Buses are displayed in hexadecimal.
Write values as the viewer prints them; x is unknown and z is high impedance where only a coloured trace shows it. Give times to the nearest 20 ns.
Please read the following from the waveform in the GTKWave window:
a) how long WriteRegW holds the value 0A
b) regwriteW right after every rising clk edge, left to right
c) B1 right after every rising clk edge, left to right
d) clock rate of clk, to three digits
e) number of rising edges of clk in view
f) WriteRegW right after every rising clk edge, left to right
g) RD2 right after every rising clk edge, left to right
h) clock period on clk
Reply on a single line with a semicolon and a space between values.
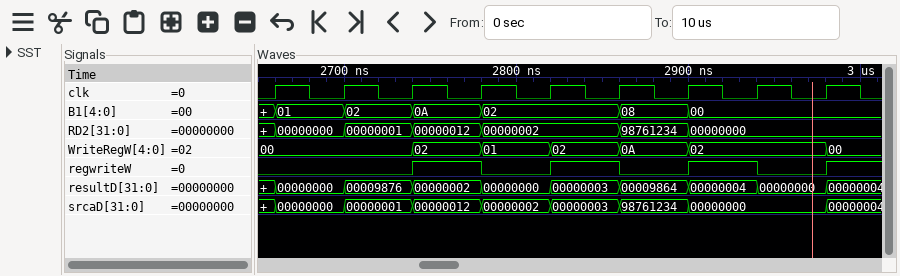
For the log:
40 ns; 0 0 1 0 1 0 1 0 1; 01, 02, 0A, 02, 02, 08, 00, 00, 00; 25.0 MHz; 9; 00, 00, 02, 01, 02, 0A, 02, 02, 00; 00000000, 00000001, 00000012, 00000002, 00000002, 98761234, 00000000, 00000000, 00000000; 40 ns
